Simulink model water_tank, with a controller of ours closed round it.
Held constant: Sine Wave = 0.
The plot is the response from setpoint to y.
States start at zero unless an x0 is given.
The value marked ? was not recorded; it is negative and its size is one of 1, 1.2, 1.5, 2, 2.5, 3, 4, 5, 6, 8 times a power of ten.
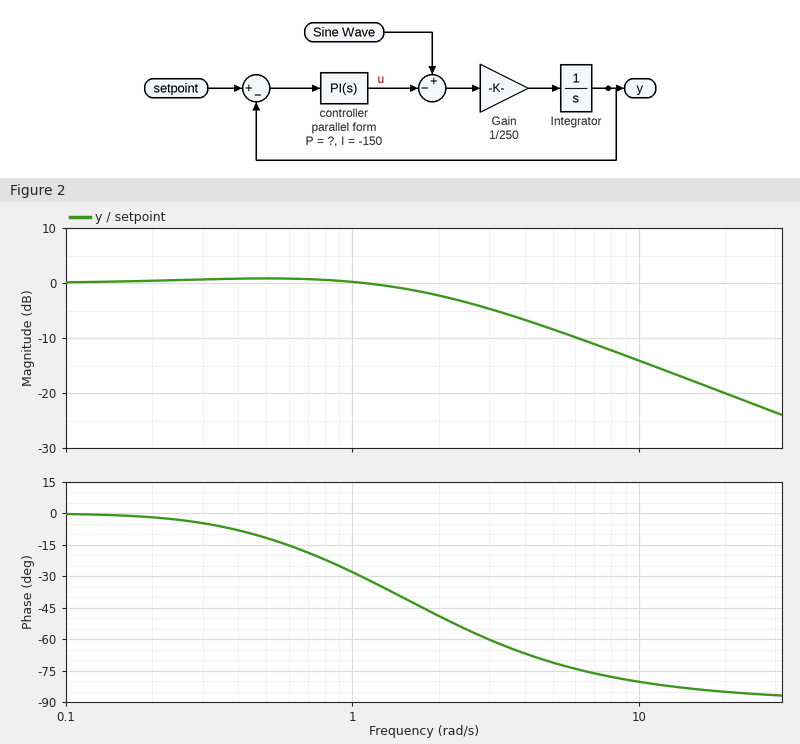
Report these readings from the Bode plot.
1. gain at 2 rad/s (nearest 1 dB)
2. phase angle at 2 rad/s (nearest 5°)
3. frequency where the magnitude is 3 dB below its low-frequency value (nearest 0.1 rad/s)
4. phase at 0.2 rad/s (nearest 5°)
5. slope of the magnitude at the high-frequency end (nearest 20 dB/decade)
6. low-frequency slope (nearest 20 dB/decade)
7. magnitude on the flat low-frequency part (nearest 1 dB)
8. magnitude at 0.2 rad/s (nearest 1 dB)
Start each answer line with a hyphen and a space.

- -2 dB
- -50°
- 2.2 rad/s
- 0°
- -20 dB/decade
- 0 dB/decade
- 0 dB
- 0 dB
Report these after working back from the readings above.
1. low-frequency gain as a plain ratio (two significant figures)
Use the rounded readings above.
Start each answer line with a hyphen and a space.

- 1.0
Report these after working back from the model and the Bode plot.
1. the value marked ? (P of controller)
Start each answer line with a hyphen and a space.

- -500
